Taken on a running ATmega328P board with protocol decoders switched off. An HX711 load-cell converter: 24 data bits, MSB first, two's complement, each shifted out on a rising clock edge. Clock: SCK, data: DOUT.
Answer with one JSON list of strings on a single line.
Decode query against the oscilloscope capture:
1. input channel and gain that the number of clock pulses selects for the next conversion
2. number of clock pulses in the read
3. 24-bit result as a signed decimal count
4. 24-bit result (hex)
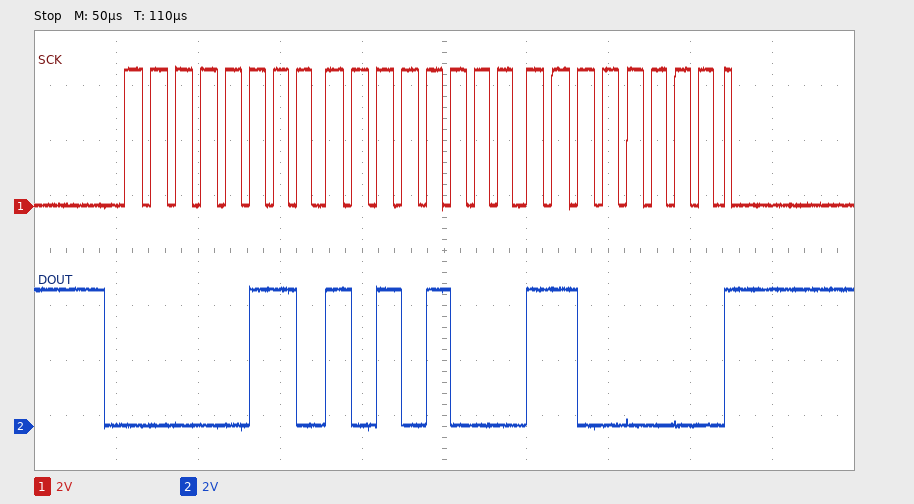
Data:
["channel A, gain 128", "25", "436416", "0x06A8C0"]
